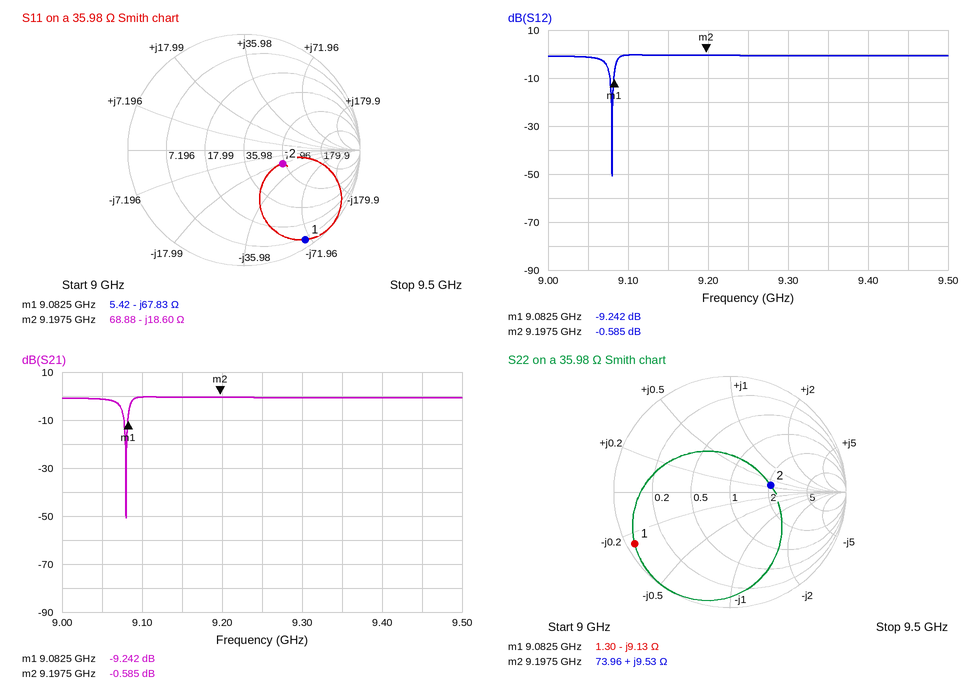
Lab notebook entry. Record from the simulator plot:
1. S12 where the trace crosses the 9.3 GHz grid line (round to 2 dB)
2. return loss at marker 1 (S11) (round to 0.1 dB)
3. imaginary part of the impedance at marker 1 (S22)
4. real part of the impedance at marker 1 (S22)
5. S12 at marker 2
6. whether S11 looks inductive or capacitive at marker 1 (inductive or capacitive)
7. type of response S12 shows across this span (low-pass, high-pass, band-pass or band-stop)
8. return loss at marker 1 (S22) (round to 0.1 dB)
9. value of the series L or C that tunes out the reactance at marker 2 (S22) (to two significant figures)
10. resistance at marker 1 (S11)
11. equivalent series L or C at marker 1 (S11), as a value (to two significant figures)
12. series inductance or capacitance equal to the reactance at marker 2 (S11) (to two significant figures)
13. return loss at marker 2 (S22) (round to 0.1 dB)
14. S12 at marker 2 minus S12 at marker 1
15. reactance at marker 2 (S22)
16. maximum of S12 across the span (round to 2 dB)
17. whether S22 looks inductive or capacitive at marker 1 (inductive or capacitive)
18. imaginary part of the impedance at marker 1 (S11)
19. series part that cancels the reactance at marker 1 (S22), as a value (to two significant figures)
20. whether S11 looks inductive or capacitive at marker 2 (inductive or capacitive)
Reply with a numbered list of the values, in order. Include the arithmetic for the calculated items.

1. 0 dB
2. 0.6 dB
3. -9.13 Ω
4. 1.30 Ω
5. -0.585 dB
6. capacitive
7. band-stop
8. 0.6 dB
9. C = 1/(2π × 9.1975 GHz × 9.53 Ω) ≈ 1.8 pF
10. 5.42 Ω
11. C = 1/(2π × 9.0825 GHz × 67.83 Ω) ≈ 258 fF, so 260 fF to two significant figures
12. C = 1/(2π × 9.1975 GHz × 18.6 Ω) ≈ 930 fF
13. 9.0 dB
14. -0.585 − (-9.242) = 8.657 dB
15. +9.53 Ω
16. 0 dB
17. capacitive
18. -67.83 Ω
19. L = 9.13 Ω/(2π × 9.0825 GHz) ≈ 160 pH
20. capacitive
